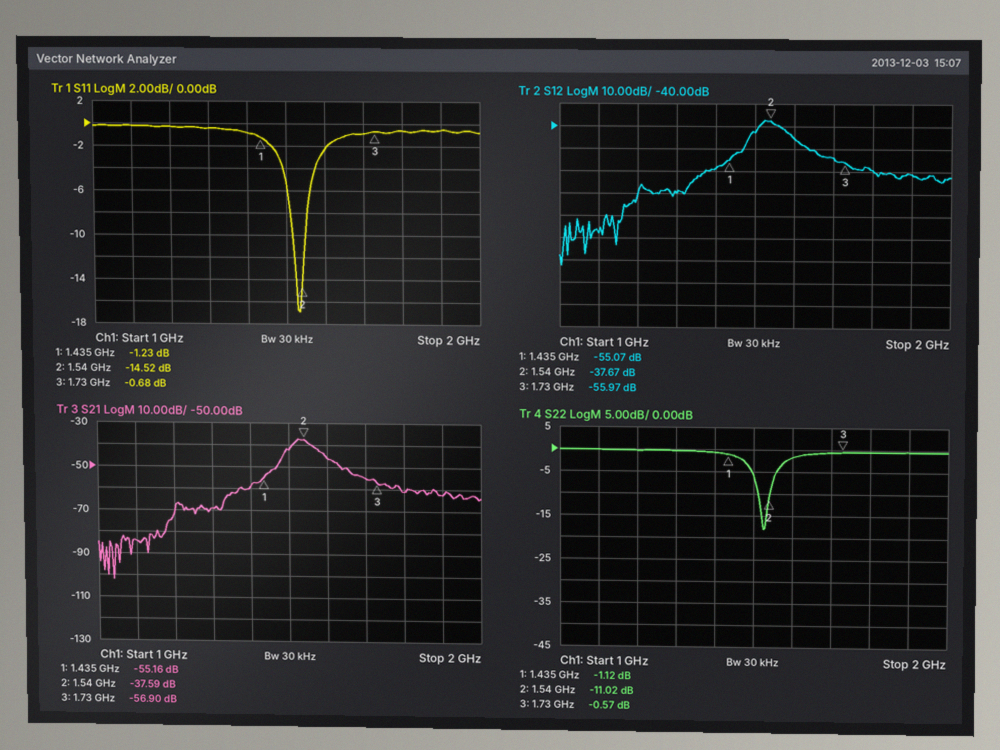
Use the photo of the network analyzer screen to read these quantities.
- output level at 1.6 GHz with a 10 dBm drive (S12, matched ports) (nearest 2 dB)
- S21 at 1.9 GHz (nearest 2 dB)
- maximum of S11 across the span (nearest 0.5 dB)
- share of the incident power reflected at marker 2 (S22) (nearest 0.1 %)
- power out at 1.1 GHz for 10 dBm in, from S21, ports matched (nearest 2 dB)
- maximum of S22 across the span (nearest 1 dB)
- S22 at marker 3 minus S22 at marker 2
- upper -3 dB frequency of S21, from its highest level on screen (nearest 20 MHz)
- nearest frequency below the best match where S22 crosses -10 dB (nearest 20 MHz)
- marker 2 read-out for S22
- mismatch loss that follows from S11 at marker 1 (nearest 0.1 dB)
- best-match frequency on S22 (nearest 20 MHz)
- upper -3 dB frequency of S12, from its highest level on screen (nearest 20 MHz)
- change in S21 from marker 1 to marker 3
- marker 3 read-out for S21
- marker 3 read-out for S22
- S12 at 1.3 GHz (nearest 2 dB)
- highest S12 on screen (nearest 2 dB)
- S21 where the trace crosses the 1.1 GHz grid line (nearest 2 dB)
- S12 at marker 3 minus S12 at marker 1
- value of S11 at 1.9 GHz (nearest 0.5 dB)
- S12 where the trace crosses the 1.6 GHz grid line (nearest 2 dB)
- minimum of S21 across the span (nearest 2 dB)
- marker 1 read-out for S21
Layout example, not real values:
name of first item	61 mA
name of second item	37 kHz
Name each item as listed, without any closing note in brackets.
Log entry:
output level at 1.6 GHz with a 10 dBm drive (S12, matched ports)	-36 dBm
S21 at 1.9 GHz	-62 dB
maximum of S11 across the span	0.0 dB
share of the incident power reflected at marker 2 (S22)	7.9 %
power out at 1.1 GHz for 10 dBm in, from S21, ports matched	-74 dBm
maximum of S22 across the span	0 dB
S22 at marker 3 minus S22 at marker 2	10.45 dB
upper -3 dB frequency of S21, from its highest level on screen	1.56 GHz
nearest frequency below the best match where S22 crosses -10 dB	1.52 GHz
marker 2 read-out for S22	-11.02 dB
mismatch loss that follows from S11 at marker 1	6.1 dB
best-match frequency on S22	1.52 GHz
upper -3 dB frequency of S12, from its highest level on screen	1.56 GHz
change in S21 from marker 1 to marker 3	-1.74 dB
marker 3 read-out for S21	-56.90 dB
marker 3 read-out for S22	-0.57 dB
S12 at 1.3 GHz	-70 dB
highest S12 on screen	-38 dB
S21 where the trace crosses the 1.1 GHz grid line	-84 dB
S12 at marker 3 minus S12 at marker 1	-0.90 dB
value of S11 at 1.9 GHz	-0.5 dB
S12 where the trace crosses the 1.6 GHz grid line	-46 dB
minimum of S21 across the span	-102 dB
marker 1 read-out for S21	-55.16 dB
